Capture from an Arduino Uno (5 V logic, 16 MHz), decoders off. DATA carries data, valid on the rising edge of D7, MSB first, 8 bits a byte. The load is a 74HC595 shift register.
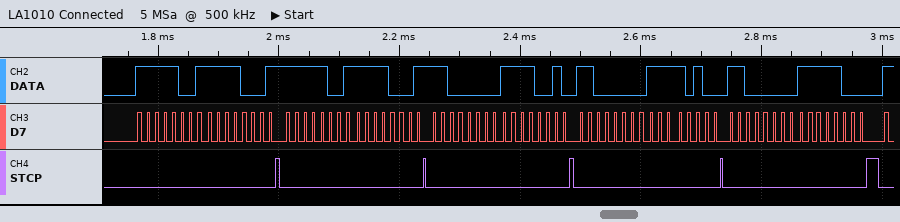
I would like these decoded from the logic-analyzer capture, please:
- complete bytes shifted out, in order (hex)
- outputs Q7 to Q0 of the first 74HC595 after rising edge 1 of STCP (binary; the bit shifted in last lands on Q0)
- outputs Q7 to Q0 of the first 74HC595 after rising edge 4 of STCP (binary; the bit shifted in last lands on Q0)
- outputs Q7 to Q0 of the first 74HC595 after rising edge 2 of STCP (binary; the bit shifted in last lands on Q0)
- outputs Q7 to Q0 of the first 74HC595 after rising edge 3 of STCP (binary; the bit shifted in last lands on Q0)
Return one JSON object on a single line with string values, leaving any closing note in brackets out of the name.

{"complete bytes shifted out, in order": "F9 F1 F9 F1 C0 F2 C0 F4 C0 F8", "outputs Q7 to Q0 of the first 74HC595 after rising edge 1 of STCP": "11110001", "outputs Q7 to Q0 of the first 74HC595 after rising edge 4 of STCP": "11110100", "outputs Q7 to Q0 of the first 74HC595 after rising edge 2 of STCP": "11110001", "outputs Q7 to Q0 of the first 74HC595 after rising edge 3 of STCP": "11110010"}
